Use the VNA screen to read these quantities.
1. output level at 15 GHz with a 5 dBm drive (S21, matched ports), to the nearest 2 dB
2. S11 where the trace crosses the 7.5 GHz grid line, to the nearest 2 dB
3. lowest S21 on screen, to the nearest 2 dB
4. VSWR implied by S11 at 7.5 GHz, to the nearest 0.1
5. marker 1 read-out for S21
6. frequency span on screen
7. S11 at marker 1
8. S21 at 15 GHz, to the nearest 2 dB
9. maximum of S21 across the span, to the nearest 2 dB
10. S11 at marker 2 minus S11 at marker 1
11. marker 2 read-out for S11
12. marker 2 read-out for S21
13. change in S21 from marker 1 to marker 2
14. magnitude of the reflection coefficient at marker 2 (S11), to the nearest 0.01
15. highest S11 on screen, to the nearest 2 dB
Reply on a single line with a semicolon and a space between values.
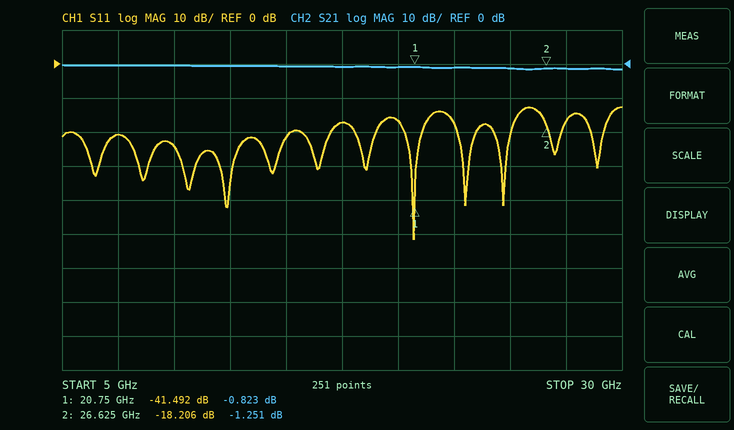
4 dBm; -20 dB; -2 dB; 1.2; -0.823 dB; 25 GHz; -41.492 dB; 0 dB; 0 dB; 23.286 dB; -18.206 dB; -1.251 dB; -0.428 dB; 0.12; -12 dB
